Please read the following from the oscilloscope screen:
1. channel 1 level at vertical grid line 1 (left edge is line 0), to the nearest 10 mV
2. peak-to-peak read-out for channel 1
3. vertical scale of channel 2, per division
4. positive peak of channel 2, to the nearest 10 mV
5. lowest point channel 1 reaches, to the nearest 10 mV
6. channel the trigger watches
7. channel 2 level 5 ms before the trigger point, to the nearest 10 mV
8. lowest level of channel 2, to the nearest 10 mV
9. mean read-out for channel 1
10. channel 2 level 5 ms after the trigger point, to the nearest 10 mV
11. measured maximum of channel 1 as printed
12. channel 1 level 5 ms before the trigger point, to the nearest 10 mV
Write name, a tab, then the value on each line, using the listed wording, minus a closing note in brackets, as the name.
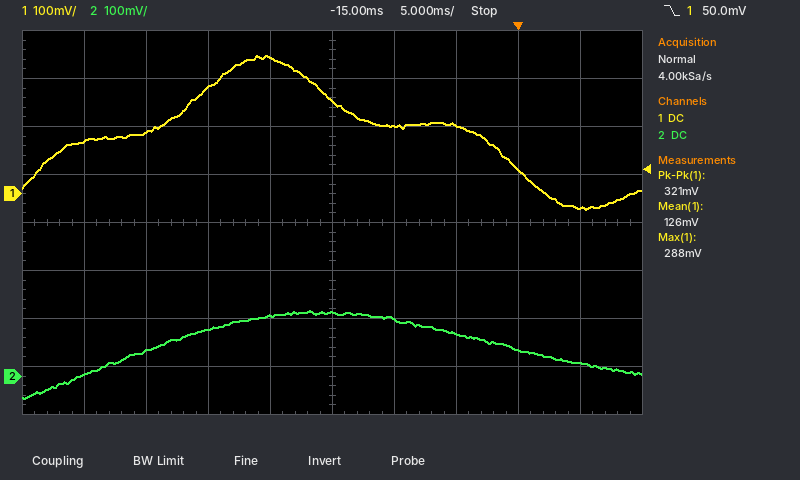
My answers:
channel 1 level at vertical grid line 1 (left edge is line 0), to the nearest 10 mV	110 mV
peak-to-peak read-out for channel 1	321 mV
vertical scale of channel 2, per division	100 mV
positive peak of channel 2, to the nearest 10 mV	140 mV
lowest point channel 1 reaches, to the nearest 10 mV	-30 mV
channel the trigger watches	channel 1
channel 2 level 5 ms before the trigger point, to the nearest 10 mV	90 mV
lowest level of channel 2, to the nearest 10 mV	-50 mV
mean read-out for channel 1	126 mV
channel 2 level 5 ms after the trigger point, to the nearest 10 mV	30 mV
measured maximum of channel 1 as printed	288 mV
channel 1 level 5 ms before the trigger point, to the nearest 10 mV	140 mV
